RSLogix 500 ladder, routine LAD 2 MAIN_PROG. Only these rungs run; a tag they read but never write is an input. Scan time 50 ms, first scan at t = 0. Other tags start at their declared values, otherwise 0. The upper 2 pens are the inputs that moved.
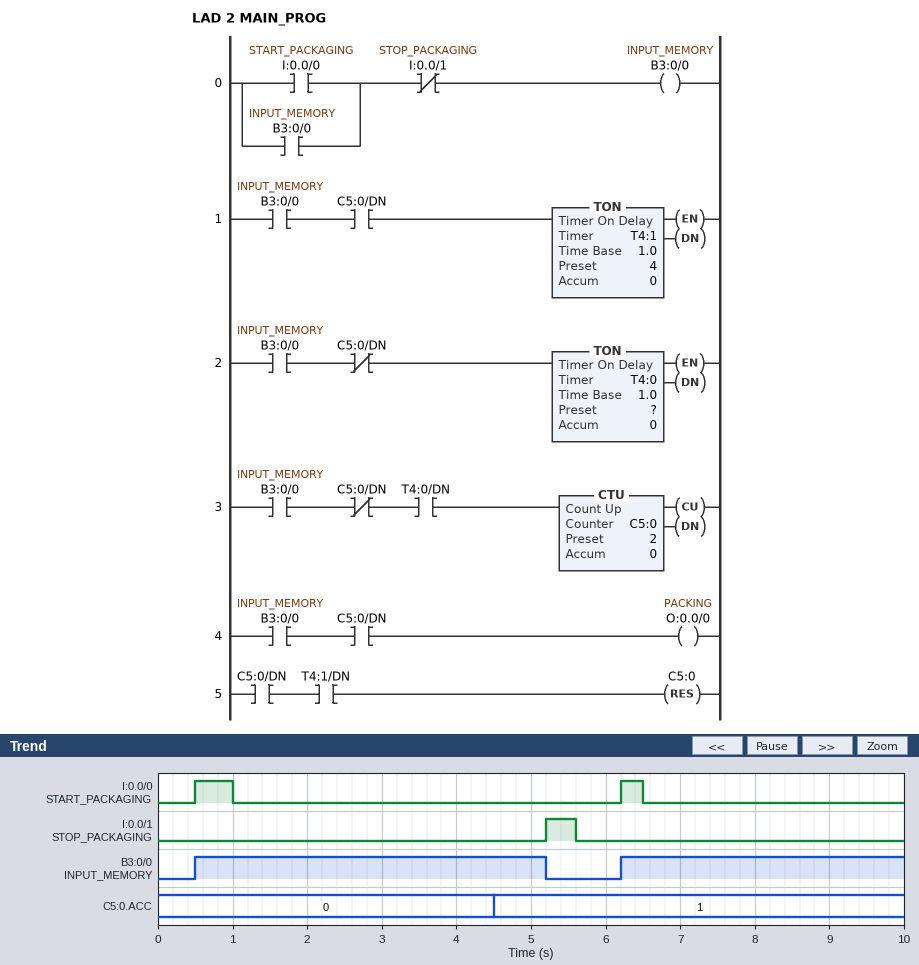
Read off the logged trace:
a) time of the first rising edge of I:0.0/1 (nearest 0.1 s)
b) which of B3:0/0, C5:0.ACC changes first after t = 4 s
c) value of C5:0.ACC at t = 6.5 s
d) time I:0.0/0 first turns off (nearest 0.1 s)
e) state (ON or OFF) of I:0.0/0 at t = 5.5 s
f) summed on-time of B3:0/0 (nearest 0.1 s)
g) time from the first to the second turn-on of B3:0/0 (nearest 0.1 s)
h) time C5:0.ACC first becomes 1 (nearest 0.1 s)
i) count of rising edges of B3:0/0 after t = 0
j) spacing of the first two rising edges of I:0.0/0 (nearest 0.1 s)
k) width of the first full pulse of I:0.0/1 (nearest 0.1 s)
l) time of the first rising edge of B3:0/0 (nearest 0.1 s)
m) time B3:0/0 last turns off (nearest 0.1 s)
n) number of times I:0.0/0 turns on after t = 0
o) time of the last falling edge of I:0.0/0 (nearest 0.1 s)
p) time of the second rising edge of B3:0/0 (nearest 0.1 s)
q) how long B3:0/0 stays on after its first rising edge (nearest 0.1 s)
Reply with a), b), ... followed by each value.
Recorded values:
a) 5.2 s
b) C5:0.ACC
c) 1
d) 1.0 s
e) OFF
f) 8.5 s
g) 5.7 s
h) 4.5 s
i) 2
j) 5.7 s
k) 0.4 s
l) 0.5 s
m) 5.2 s
n) 2
o) 6.5 s
p) 6.2 s
q) 4.7 s
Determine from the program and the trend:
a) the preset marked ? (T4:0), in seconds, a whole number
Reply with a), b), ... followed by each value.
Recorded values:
a) 4 s
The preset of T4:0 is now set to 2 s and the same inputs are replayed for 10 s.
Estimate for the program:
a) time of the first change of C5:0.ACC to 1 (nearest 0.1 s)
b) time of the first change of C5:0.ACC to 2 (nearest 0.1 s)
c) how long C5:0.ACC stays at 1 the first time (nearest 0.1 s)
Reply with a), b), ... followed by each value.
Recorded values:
a) 2.5 s
b) 8.2 s
c) 5.7 s
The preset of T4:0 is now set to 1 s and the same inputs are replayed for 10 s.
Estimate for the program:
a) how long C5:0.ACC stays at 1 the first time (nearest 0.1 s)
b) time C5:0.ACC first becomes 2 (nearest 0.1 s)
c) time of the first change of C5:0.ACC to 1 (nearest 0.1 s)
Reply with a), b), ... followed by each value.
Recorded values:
a) 5.7 s
b) 7.2 s
c) 1.5 s
